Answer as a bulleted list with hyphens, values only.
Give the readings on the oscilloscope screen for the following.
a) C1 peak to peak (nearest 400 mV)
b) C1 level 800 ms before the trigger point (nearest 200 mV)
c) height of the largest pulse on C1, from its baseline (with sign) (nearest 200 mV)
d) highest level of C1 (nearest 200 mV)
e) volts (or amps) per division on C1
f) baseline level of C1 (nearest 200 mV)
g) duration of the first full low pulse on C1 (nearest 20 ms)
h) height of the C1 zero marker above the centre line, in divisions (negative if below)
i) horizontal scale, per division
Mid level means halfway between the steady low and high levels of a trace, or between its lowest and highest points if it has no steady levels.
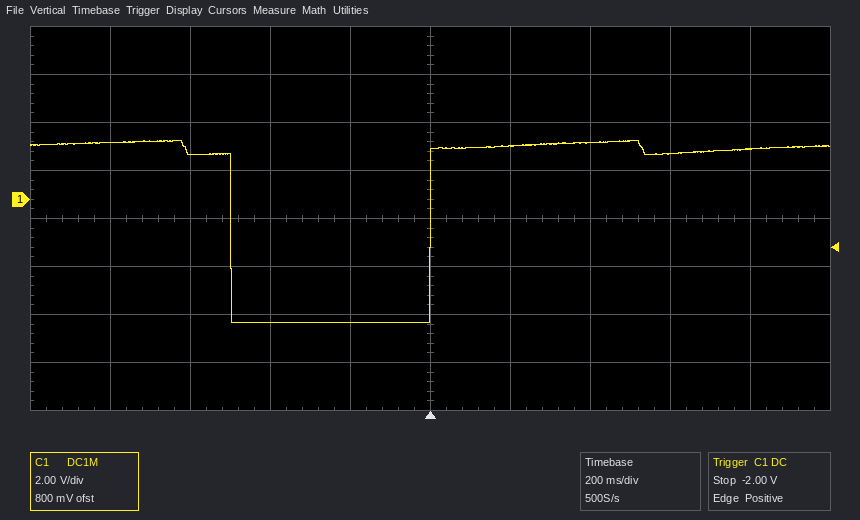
- 7.6 V
- 2.4 V
- -7.4 V
- 2.4 V
- 2 V
- 2.2 V
- 500 ms
- +0.4 div
- 200 ms
